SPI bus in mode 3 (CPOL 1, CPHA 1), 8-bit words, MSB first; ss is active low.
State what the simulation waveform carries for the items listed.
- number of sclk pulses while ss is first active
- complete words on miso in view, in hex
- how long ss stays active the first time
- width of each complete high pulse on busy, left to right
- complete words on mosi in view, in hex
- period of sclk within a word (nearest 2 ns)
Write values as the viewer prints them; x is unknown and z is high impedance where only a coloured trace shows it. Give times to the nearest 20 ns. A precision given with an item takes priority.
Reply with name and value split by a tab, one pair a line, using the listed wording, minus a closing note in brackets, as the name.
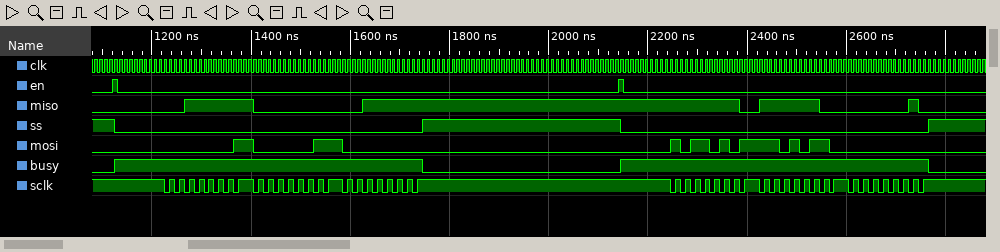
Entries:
number of sclk pulses while ss is first active	24
complete words on miso in view, in hex	3F, 00, 3F, FE, FC, 02
how long ss stays active the first time	620 ns
width of each complete high pulse on busy, left to right	620 ns, 620 ns
complete words on mosi in view, in hex	01, 03, 00, B5, D6, 00
period of sclk within a word	20 ns
